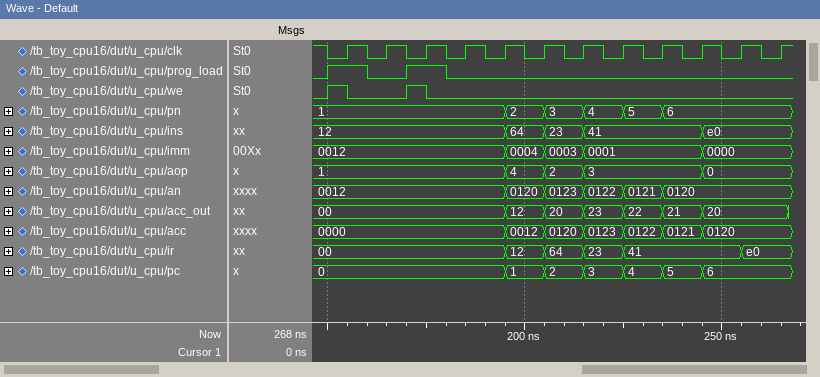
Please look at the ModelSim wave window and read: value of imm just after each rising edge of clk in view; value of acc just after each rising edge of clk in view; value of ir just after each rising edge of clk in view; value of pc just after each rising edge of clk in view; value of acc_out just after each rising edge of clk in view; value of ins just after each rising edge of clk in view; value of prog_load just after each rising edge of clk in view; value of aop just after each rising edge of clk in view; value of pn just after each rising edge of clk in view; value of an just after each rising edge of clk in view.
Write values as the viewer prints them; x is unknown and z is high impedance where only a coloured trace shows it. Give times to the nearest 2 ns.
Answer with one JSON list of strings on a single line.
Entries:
["0012, 0012, 0012, 0012, 0004, 0003, 0001, 0001, 0001, 0000, 0000, 0000", "0000, 0000, 0000, 0000, 0012, 0120, 0123, 0122, 0121, 0120, 0120, 0120", "00, 00, 00, 00, 12, 64, 23, 41, 41, 41, e0, e0", "0, 0, 0, 0, 1, 2, 3, 4, 5, 6, 6, 6", "00, 00, 00, 00, 12, 20, 23, 22, 21, 20, 20, 20", "12, 12, 12, 12, 64, 23, 41, 41, 41, e0, e0, e0", "1 0 1 0 0 0 0 0 0 0 0 0", "1, 1, 1, 1, 4, 2, 3, 3, 3, 0, 0, 0", "1, 1, 1, 1, 2, 3, 4, 5, 6, 6, 6, 6", "0012, 0012, 0012, 0012, 0120, 0123, 0122, 0121, 0120, 0120, 0120, 0120"]
